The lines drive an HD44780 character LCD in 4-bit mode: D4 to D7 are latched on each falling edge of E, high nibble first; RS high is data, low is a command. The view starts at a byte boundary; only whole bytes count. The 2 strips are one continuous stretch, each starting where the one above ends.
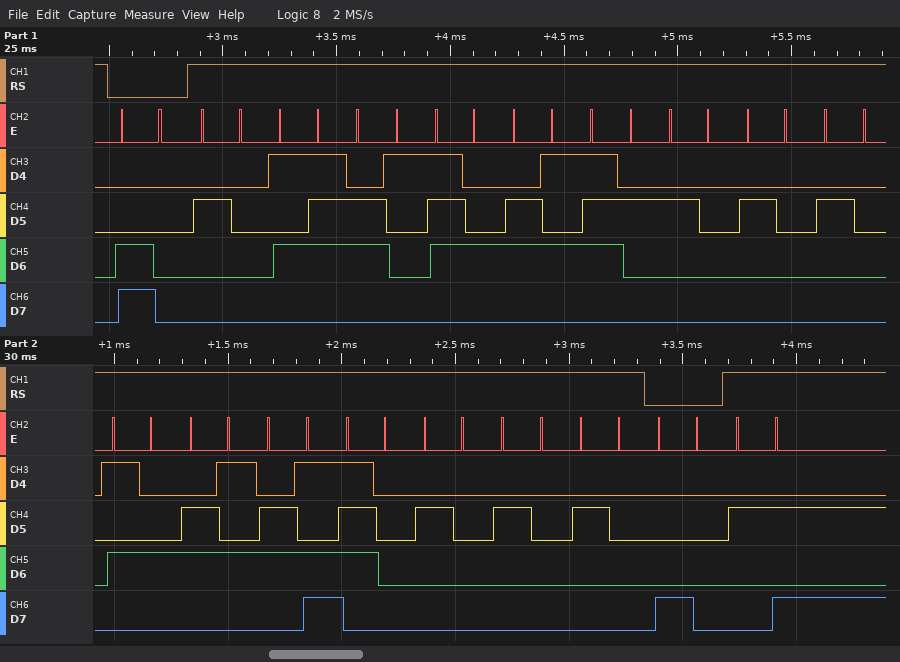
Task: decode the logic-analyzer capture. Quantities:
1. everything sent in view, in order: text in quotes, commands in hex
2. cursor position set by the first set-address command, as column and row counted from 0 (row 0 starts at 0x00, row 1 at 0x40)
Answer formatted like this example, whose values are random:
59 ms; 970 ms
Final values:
0xC0 " Water   Temp   " 0x80 "*"; column 0, row 1
